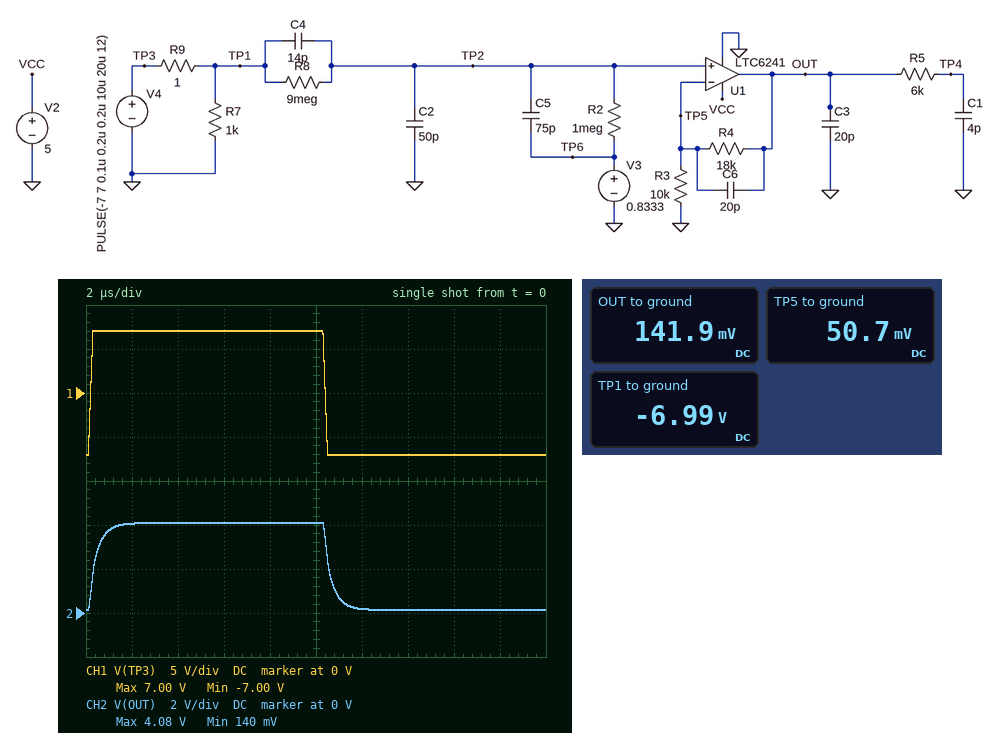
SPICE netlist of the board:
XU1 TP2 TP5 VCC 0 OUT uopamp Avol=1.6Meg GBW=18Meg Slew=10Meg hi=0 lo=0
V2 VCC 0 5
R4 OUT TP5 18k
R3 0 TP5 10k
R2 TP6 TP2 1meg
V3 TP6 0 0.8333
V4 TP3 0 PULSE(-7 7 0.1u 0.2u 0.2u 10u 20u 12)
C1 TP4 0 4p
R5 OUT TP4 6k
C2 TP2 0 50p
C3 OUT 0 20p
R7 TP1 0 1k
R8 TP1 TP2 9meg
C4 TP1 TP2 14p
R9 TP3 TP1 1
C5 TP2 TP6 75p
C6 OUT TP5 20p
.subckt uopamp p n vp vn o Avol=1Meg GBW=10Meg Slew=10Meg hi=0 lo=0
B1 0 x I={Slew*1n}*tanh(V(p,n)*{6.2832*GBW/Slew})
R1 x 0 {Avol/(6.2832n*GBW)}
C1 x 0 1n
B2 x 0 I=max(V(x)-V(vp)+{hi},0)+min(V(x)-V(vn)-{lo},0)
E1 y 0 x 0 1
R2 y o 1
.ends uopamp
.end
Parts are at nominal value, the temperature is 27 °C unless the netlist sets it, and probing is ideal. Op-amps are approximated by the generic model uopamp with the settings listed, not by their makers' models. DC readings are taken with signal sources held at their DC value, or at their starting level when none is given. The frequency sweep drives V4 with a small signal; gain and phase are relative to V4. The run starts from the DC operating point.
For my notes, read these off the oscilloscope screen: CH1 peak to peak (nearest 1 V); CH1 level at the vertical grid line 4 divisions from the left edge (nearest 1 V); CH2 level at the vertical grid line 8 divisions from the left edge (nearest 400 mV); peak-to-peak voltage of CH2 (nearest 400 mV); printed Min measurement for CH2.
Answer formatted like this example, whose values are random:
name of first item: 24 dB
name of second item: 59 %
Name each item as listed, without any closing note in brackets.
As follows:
CH1 peak to peak: 14 V
CH1 level at the vertical grid line 4 divisions from the left edge: 7 V
CH2 level at the vertical grid line 8 divisions from the left edge: 0 V
peak-to-peak voltage of CH2: 4.0 V
printed Min measurement for CH2: 140 mV
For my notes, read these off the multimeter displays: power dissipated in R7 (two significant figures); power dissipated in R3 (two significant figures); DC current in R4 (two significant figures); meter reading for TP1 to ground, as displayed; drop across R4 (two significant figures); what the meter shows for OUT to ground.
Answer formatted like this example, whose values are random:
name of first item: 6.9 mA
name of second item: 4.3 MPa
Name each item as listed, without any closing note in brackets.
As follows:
power dissipated in R7: 49 mW
power dissipated in R3: 260 nW
DC current in R4: 5.1 µA
meter reading for TP1 to ground, as displayed: -6.99 V
drop across R4: 91 mV
what the meter shows for OUT to ground: 141.9 mV
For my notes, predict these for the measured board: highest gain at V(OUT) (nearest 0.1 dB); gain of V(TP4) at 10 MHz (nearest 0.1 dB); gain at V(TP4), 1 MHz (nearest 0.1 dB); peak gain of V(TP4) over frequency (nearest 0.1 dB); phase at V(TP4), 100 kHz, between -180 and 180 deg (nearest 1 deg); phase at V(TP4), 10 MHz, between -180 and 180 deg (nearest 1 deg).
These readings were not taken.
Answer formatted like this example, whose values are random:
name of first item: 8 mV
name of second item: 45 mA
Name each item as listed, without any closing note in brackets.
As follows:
highest gain at V(OUT): -11.0 dB
gain of V(TP4) at 10 MHz: -26.5 dB
gain at V(TP4), 1 MHz: -17.1 dB
peak gain of V(TP4) over frequency: -11.0 dB
phase at V(TP4), 100 kHz, between -180 and 180 deg: -10 deg
phase at V(TP4), 10 MHz, between -180 and 180 deg: -89 deg
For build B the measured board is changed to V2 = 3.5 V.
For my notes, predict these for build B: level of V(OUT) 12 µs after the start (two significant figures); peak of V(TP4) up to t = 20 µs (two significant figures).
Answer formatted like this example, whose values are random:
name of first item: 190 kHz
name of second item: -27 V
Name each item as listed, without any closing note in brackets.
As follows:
level of V(OUT) 12 µs after the start: 170 mV
peak of V(TP4) up to t = 20 µs: 3.5 V
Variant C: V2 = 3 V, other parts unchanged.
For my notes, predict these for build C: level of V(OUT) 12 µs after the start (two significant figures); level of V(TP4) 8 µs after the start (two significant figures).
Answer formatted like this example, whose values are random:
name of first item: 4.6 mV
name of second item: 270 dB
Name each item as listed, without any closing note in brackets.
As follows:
level of V(OUT) 12 µs after the start: 170 mV
level of V(TP4) 8 µs after the start: 3.0 V
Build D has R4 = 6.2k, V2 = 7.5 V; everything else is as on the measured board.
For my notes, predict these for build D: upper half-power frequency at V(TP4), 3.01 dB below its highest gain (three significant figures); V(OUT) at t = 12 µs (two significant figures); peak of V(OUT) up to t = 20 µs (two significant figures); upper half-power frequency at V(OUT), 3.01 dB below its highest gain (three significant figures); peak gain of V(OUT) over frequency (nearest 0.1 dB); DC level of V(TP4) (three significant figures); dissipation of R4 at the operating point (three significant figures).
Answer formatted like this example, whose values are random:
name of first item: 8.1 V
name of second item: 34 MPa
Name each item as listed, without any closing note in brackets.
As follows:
upper half-power frequency at V(TP4), 3.01 dB below its highest gain: 1.86 MHz
V(OUT) at t = 12 µs: 81 mV
peak of V(OUT) up to t = 20 µs: 2.4 V
upper half-power frequency at V(OUT), 3.01 dB below its highest gain: 2.16 MHz
peak gain of V(OUT) over frequency: -15.8 dB
DC level of V(TP4): 82.1 mV
dissipation of R4 at the operating point: 159 nW
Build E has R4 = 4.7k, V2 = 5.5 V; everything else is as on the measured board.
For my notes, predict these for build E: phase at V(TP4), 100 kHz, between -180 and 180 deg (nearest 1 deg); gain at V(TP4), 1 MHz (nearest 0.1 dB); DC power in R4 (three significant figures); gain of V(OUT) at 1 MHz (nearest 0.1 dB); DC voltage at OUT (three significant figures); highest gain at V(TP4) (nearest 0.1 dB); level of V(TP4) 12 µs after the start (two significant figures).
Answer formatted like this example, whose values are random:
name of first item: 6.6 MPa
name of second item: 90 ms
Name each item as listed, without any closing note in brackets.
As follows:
phase at V(TP4), 100 kHz, between -180 and 180 deg: -2 deg
gain at V(TP4), 1 MHz: -17.5 dB
DC power in R4: 121 nW
gain of V(OUT) at 1 MHz: -17.4 dB
DC voltage at OUT: 74.5 mV
highest gain at V(TP4): -16.6 dB
level of V(TP4) 12 µs after the start: 73 mV
